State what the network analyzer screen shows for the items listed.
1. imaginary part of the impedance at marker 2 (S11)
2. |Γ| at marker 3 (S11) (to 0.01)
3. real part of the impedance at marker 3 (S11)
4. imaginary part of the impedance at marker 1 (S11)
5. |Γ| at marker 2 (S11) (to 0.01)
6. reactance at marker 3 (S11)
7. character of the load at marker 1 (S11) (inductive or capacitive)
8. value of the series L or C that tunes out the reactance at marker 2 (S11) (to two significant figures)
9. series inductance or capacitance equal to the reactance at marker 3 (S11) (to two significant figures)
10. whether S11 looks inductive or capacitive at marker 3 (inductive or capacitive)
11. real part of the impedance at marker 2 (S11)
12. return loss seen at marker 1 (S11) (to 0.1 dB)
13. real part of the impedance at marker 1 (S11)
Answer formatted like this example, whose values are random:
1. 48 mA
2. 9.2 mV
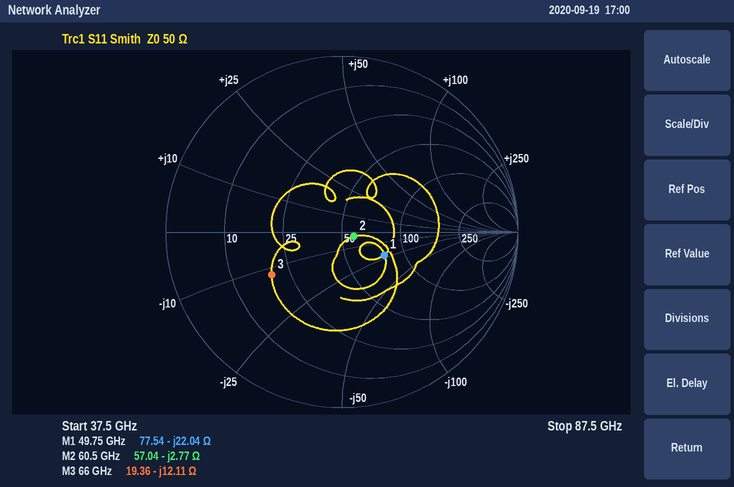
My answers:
1. -2.77 Ω
2. 0.47
3. 19.36 Ω
4. -22.04 Ω
5. 0.07
6. -12.11 Ω
7. capacitive
8. 7.3 pH
9. 200 fF
10. capacitive
11. 57.04 Ω
12. 11.3 dB
13. 77.54 Ω
